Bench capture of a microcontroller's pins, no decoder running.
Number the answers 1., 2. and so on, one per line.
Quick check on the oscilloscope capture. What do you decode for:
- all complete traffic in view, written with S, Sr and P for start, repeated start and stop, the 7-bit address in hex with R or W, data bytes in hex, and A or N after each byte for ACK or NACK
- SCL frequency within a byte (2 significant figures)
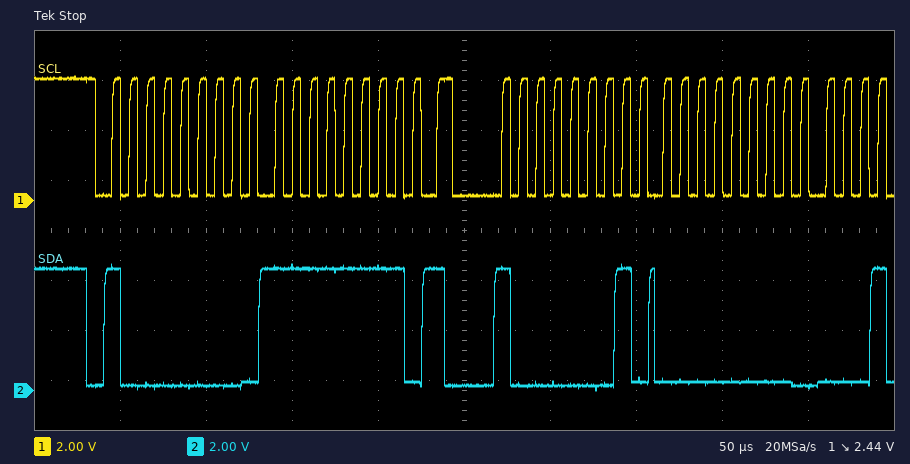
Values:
1. S 40W A FF A Sr 40R A 00 A
2. 100 kHz
